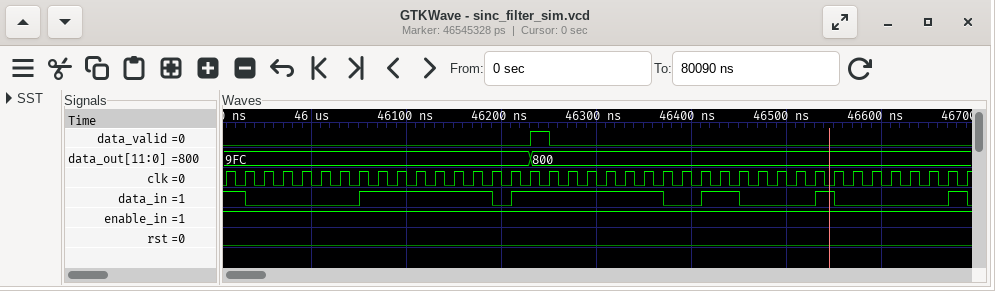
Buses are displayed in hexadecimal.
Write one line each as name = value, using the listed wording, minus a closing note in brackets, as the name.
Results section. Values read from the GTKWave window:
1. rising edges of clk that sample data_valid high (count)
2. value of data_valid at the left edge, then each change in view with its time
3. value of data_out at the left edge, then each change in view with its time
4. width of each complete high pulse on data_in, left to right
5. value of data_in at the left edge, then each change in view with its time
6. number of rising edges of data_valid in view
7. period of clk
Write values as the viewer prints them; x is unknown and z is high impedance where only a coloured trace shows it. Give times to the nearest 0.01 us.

rising edges of clk that sample data_valid high = 1
value of data_valid at the left edge, then each change in view with its time = 0, 1 at 46.23 us, 0 at 46.25 us
value of data_out at the left edge, then each change in view with its time = 9FC, 800 at 46.23 us
width of each complete high pulse on data_in, left to right = 0.14 us, 0.16 us, 0.04 us, 0.02 us, 0.02 us
value of data_in at the left edge, then each change in view with its time = 1, 0 at 45.93 us, 1 at 46.05 us, 0 at 46.19 us, 1 at 46.21 us, 0 at 46.37 us, 1 at 46.41 us, 0 at 46.45 us, 1 at 46.53 us, 0 at 46.55 us, 1 at 46.67 us, 0 at 46.69 us
number of rising edges of data_valid in view = 1
period of clk = 0.02 us
